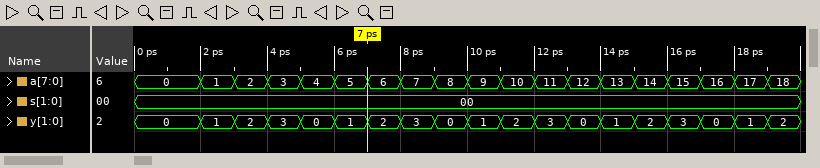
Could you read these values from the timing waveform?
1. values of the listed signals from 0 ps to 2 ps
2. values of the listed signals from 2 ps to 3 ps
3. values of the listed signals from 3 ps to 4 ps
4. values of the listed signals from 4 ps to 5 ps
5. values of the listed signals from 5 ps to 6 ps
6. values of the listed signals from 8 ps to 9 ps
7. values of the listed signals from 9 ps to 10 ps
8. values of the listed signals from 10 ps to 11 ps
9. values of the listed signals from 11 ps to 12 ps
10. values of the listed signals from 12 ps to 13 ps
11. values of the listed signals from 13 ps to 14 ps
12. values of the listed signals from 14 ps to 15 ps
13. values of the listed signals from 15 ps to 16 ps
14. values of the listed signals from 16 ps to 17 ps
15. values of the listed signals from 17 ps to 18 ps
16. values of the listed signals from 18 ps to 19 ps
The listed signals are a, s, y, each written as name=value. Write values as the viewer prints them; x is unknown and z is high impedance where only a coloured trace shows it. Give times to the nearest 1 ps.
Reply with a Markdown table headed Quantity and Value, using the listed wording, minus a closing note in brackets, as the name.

| Quantity | Value |
|---|---|
| values of the listed signals from 0 ps to 2 ps | a=0, s=00, y=0 |
| values of the listed signals from 2 ps to 3 ps | a=1, s=00, y=1 |
| values of the listed signals from 3 ps to 4 ps | a=2, s=00, y=2 |
| values of the listed signals from 4 ps to 5 ps | a=3, s=00, y=3 |
| values of the listed signals from 5 ps to 6 ps | a=4, s=00, y=0 |
| values of the listed signals from 8 ps to 9 ps | a=7, s=00, y=3 |
| values of the listed signals from 9 ps to 10 ps | a=8, s=00, y=0 |
| values of the listed signals from 10 ps to 11 ps | a=9, s=00, y=1 |
| values of the listed signals from 11 ps to 12 ps | a=10, s=00, y=2 |
| values of the listed signals from 12 ps to 13 ps | a=11, s=00, y=3 |
| values of the listed signals from 13 ps to 14 ps | a=12, s=00, y=0 |
| values of the listed signals from 14 ps to 15 ps | a=13, s=00, y=1 |
| values of the listed signals from 15 ps to 16 ps | a=14, s=00, y=2 |
| values of the listed signals from 16 ps to 17 ps | a=15, s=00, y=3 |
| values of the listed signals from 17 ps to 18 ps | a=16, s=00, y=0 |
| values of the listed signals from 18 ps to 19 ps | a=17, s=00, y=1 |
